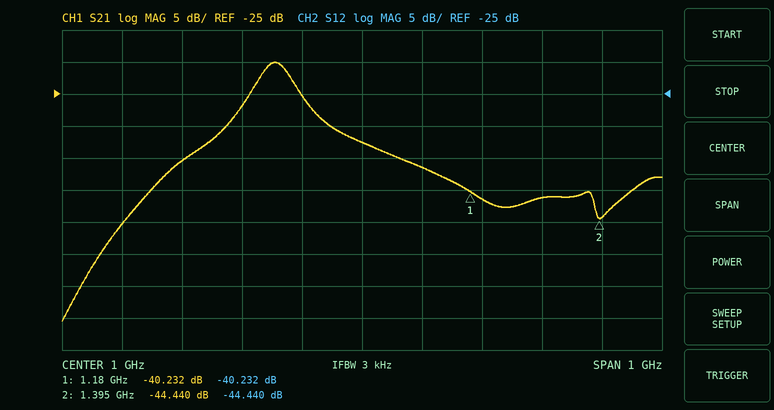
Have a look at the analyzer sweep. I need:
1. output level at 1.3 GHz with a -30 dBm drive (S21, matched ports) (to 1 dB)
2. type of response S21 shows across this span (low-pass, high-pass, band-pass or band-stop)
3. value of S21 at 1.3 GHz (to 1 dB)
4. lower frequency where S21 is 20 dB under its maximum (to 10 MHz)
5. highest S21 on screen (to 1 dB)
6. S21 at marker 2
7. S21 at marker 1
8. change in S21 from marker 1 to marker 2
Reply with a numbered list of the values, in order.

1. -71 dBm
2. band-pass
3. -41 dB
4. 650 MHz
5. -20 dB
6. -44.440 dB
7. -40.232 dB
8. -4.208 dB
